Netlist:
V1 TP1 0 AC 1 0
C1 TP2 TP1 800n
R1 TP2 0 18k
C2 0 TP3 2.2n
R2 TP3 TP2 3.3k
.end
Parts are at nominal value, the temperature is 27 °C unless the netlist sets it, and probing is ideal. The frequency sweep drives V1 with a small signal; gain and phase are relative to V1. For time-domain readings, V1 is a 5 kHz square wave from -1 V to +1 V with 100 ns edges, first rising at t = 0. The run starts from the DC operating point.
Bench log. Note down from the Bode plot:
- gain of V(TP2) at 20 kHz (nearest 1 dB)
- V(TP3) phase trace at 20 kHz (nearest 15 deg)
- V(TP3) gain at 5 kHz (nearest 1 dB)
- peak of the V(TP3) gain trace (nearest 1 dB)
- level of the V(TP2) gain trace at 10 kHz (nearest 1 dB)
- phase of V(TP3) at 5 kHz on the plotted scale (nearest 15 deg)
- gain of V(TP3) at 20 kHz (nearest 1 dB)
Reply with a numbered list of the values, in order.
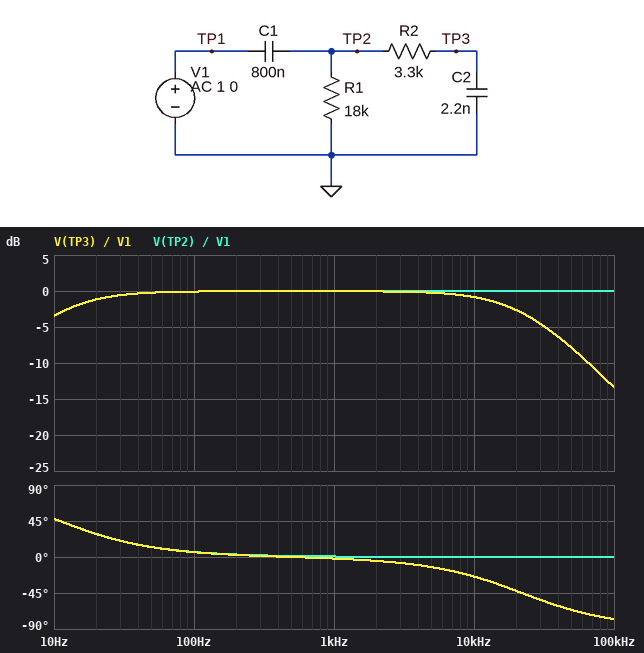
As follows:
1. 0 dB
2. -45 deg
3. 0 dB
4. 0 dB
5. 0 dB
6. -15 deg
7. -3 dB
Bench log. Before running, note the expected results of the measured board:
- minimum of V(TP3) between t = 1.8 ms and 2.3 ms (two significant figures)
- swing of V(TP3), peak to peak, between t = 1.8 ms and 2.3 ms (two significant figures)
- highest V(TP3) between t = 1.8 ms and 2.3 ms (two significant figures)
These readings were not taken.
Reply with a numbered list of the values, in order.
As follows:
1. -140 mV
2. 2.0 V
3. 1.9 V
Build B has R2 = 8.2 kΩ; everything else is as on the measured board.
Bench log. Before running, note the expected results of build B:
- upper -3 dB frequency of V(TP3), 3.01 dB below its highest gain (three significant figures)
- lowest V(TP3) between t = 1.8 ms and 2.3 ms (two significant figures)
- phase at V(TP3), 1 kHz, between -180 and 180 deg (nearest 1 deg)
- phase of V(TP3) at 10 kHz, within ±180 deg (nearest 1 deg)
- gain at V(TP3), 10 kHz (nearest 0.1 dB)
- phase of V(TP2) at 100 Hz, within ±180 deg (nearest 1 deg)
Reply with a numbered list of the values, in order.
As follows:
1. 8.87 kHz
2. -130 mV
3. -6 deg
4. -48 deg
5. -3.6 dB
6. 6 deg
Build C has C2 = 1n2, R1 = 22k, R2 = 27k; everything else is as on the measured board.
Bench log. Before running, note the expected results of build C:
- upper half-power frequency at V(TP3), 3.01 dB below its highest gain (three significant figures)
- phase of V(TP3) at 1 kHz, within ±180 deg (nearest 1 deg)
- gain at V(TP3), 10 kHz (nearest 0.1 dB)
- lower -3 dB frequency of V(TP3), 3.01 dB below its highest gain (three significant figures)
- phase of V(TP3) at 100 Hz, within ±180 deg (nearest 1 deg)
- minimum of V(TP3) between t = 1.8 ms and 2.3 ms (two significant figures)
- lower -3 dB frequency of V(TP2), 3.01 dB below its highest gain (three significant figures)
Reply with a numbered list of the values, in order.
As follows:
1. 4.94 kHz
2. -11 deg
3. -7.1 dB
4. 9.00 Hz
5. 4 deg
6. -30 mV
7. 9.06 Hz
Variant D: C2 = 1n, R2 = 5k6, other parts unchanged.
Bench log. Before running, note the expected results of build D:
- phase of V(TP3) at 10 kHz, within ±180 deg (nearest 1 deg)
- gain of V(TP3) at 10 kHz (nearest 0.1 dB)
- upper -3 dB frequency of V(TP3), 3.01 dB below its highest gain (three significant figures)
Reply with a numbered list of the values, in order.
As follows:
1. -19 deg
2. -0.5 dB
3. 28.5 kHz
